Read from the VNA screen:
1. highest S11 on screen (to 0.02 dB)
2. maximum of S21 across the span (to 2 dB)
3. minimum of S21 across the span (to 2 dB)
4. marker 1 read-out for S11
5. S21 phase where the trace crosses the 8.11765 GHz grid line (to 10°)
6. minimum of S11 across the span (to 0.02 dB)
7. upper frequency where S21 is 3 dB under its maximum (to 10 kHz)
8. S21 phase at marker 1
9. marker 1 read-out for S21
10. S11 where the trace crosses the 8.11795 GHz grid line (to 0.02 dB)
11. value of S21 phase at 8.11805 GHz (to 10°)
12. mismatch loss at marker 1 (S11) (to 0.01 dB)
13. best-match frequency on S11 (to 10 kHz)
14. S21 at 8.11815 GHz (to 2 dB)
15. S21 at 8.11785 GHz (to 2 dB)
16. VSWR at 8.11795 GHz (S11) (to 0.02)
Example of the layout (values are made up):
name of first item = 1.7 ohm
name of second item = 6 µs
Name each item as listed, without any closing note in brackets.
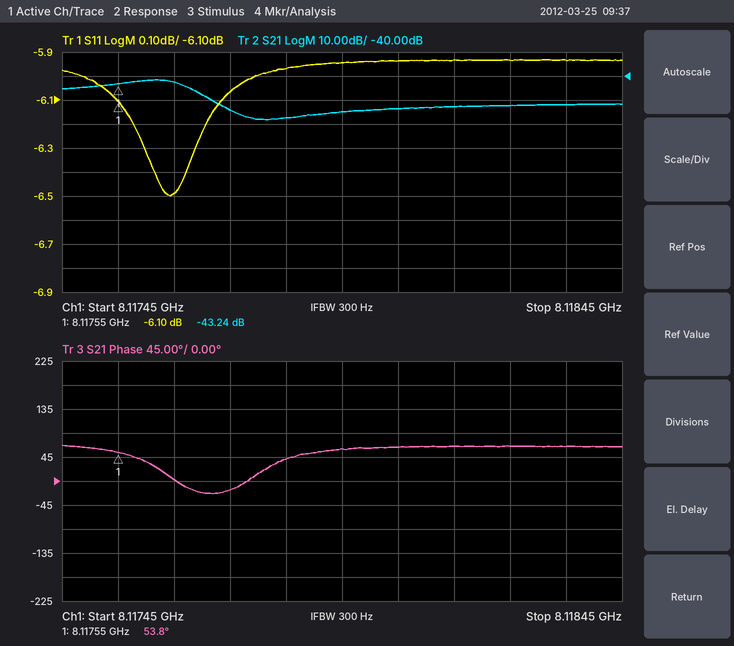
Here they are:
highest S11 on screen = -5.94 dB
maximum of S21 across the span = -42 dB
minimum of S21 across the span = -58 dB
marker 1 read-out for S11 = -6.10 dB
S21 phase where the trace crosses the 8.11765 GHz grid line = 0°
minimum of S11 across the span = -6.50 dB
upper frequency where S21 is 3 dB under its maximum = 8.11767 GHz
S21 phase at marker 1 = 53.8°
marker 1 read-out for S21 = -43.24 dB
S11 where the trace crosses the 8.11795 GHz grid line = -5.94 dB
value of S21 phase at 8.11805 GHz = 60°
mismatch loss at marker 1 (S11) = 1.22 dB
best-match frequency on S11 = 8.11764 GHz
S21 at 8.11815 GHz = -52 dB
S21 at 8.11785 GHz = -58 dB
VSWR at 8.11795 GHz (S11) = 3.04
